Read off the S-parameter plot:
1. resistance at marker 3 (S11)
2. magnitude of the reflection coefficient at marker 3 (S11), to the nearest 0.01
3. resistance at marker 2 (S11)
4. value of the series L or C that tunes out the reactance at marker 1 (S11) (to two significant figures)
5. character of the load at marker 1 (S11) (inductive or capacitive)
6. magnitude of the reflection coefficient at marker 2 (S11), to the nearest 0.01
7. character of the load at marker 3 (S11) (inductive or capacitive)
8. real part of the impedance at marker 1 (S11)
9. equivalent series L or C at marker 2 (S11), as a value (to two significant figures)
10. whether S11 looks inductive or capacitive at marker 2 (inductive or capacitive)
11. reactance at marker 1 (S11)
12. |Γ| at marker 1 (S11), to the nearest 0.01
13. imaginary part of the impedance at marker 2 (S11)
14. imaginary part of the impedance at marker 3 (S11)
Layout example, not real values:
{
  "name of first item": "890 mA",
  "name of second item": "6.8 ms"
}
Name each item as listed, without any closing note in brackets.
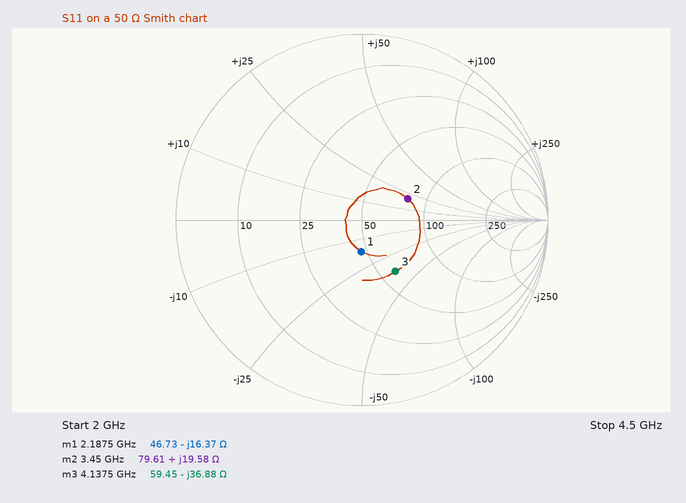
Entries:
{
  "resistance at marker 3": "59.45 Ω",
  "magnitude of the reflection coefficient at marker 3 (S11), to the nearest 0.01": "0.33",
  "resistance at marker 2": "79.61 Ω",
  "value of the series L or C that tunes out the reactance at marker 1 (S11)": "1.2 nH",
  "character of the load at marker 1 (S11)": "capacitive",
  "magnitude of the reflection coefficient at marker 2 (S11), to the nearest 0.01": "0.27",
  "character of the load at marker 3 (S11)": "capacitive",
  "real part of the impedance at marker 1": "46.73 Ω",
  "equivalent series L or C at marker 2 (S11), as a value": "900 pH",
  "whether S11 looks inductive or capacitive at marker 2": "inductive",
  "reactance at marker 1": "-16.37 Ω",
  "|Γ| at marker 1 (S11), to the nearest 0.01": "0.17",
  "imaginary part of the impedance at marker 2": "+19.58 Ω",
  "imaginary part of the impedance at marker 3": "-36.88 Ω"
}
